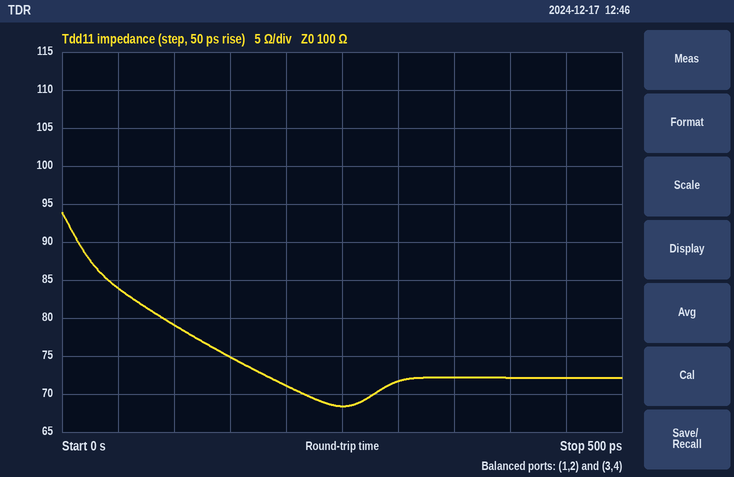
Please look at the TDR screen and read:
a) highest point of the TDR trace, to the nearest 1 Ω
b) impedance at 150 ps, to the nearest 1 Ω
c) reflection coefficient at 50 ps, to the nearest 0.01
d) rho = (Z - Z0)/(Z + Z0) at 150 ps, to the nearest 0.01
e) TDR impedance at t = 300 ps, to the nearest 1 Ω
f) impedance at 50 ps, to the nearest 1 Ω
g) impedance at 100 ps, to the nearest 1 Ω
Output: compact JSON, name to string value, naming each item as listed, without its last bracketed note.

{"highest point of the TDR trace, to the nearest 1 Ω": "94 Ω", "impedance at 150 ps, to the nearest 1 Ω": "75 Ω", "reflection coefficient at 50 ps, to the nearest 0.01": "-0.09", "rho = (Z - Z0)/(Z + Z0) at 150 ps, to the nearest 0.01": "-0.14", "TDR impedance at t = 300 ps, to the nearest 1 Ω": "72 Ω", "impedance at 50 ps, to the nearest 1 Ω": "84 Ω", "impedance at 100 ps, to the nearest 1 Ω": "79 Ω"}
